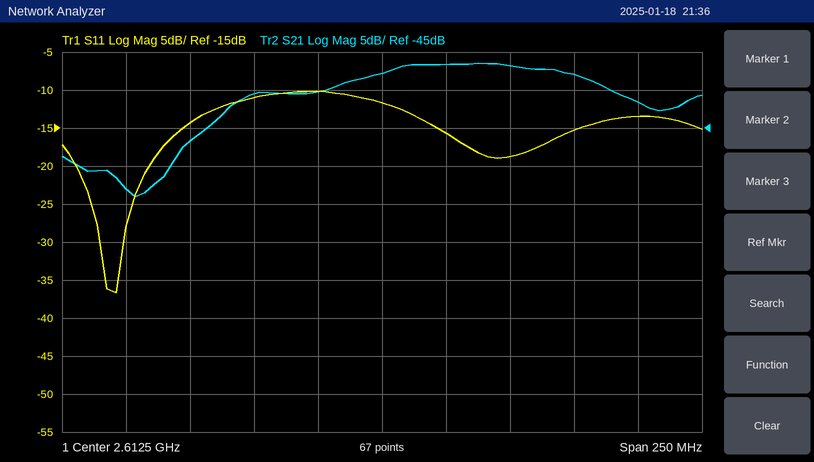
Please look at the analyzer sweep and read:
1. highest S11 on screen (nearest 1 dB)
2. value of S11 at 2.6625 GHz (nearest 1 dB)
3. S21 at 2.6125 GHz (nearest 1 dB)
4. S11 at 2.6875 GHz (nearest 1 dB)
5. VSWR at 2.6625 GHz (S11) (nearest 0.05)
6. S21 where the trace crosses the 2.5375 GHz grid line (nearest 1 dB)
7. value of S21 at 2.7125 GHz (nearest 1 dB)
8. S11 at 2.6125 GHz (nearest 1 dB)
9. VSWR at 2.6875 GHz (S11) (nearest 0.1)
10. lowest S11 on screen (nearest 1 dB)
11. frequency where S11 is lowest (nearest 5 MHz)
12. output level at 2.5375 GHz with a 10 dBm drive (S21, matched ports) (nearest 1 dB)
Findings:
-10 dB
-19 dB
-38 dB
-15 dB
1.25
-47 dB
-42 dB
-12 dB
1.4
-37 dB
2.510 GHz
-37 dBm
